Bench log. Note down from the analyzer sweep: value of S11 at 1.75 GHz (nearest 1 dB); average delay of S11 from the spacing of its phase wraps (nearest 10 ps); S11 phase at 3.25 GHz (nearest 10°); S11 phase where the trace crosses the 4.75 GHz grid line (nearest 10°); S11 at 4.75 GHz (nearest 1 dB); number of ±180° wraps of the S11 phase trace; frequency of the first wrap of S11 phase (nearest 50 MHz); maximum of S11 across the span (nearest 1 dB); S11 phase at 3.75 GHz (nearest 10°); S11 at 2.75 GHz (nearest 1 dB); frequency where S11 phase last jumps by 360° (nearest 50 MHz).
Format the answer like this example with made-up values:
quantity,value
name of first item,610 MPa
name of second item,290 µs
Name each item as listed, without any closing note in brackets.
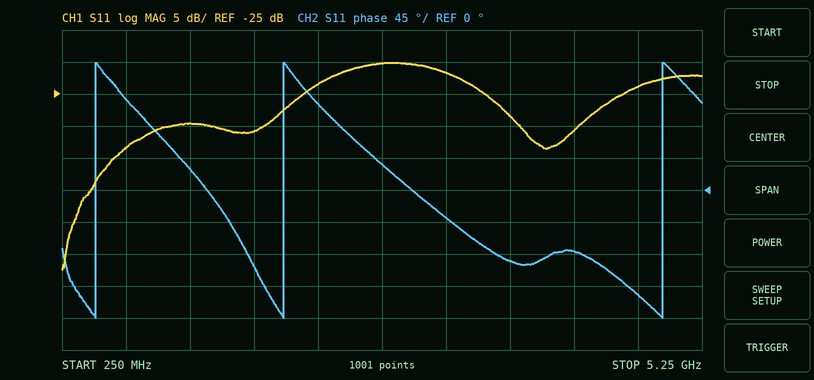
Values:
quantity,value
value of S11 at 1.75 GHz,-31 dB
average delay of S11 from the spacing of its phase wraps,450 ps
S11 phase at 3.25 GHz,-40°
S11 phase where the trace crosses the 4.75 GHz grid line,-150°
S11 at 4.75 GHz,-24 dB
number of ±180° wraps of the S11 phase trace,3
frequency of the first wrap of S11 phase,500 MHz
maximum of S11 across the span,-20 dB
S11 phase at 3.75 GHz,-100°
S11 at 2.75 GHz,-20 dB
frequency where S11 phase last jumps by 360°,4.95 GHz
